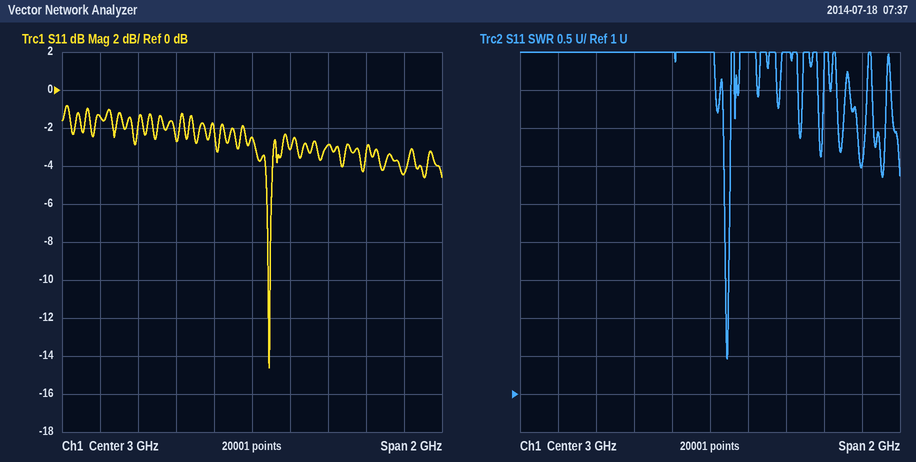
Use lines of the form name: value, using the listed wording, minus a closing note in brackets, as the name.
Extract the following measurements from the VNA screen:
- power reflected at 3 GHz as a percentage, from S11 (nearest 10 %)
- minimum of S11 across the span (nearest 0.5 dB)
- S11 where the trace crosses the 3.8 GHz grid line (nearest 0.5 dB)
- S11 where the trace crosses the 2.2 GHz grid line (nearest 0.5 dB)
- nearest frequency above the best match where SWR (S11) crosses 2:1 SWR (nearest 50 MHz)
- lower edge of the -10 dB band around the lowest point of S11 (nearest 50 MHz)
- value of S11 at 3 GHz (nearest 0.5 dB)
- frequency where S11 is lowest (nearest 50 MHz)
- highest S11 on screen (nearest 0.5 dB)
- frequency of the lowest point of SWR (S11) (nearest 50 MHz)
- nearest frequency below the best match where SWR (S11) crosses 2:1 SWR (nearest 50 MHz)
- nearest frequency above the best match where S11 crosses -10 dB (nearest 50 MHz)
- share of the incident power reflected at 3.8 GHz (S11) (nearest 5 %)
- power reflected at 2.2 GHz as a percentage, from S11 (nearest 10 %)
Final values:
power reflected at 3 GHz as a percentage, from S11: 60 %
minimum of S11 across the span: -14.5 dB
S11 where the trace crosses the 3.8 GHz grid line: -4.5 dB
S11 where the trace crosses the 2.2 GHz grid line: -1.5 dB
nearest frequency above the best match where SWR (S11) crosses 2:1 SWR: 3.10 GHz
lower edge of the -10 dB band around the lowest point of S11: 3.10 GHz
value of S11 at 3 GHz: -2.5 dB
frequency where S11 is lowest: 3.10 GHz
highest S11 on screen: -1.0 dB
frequency of the lowest point of SWR (S11): 3.10 GHz
nearest frequency below the best match where SWR (S11) crosses 2:1 SWR: 3.10 GHz
nearest frequency above the best match where S11 crosses -10 dB: 3.10 GHz
share of the incident power reflected at 3.8 GHz (S11): 35 %
power reflected at 2.2 GHz as a percentage, from S11: 70 %
